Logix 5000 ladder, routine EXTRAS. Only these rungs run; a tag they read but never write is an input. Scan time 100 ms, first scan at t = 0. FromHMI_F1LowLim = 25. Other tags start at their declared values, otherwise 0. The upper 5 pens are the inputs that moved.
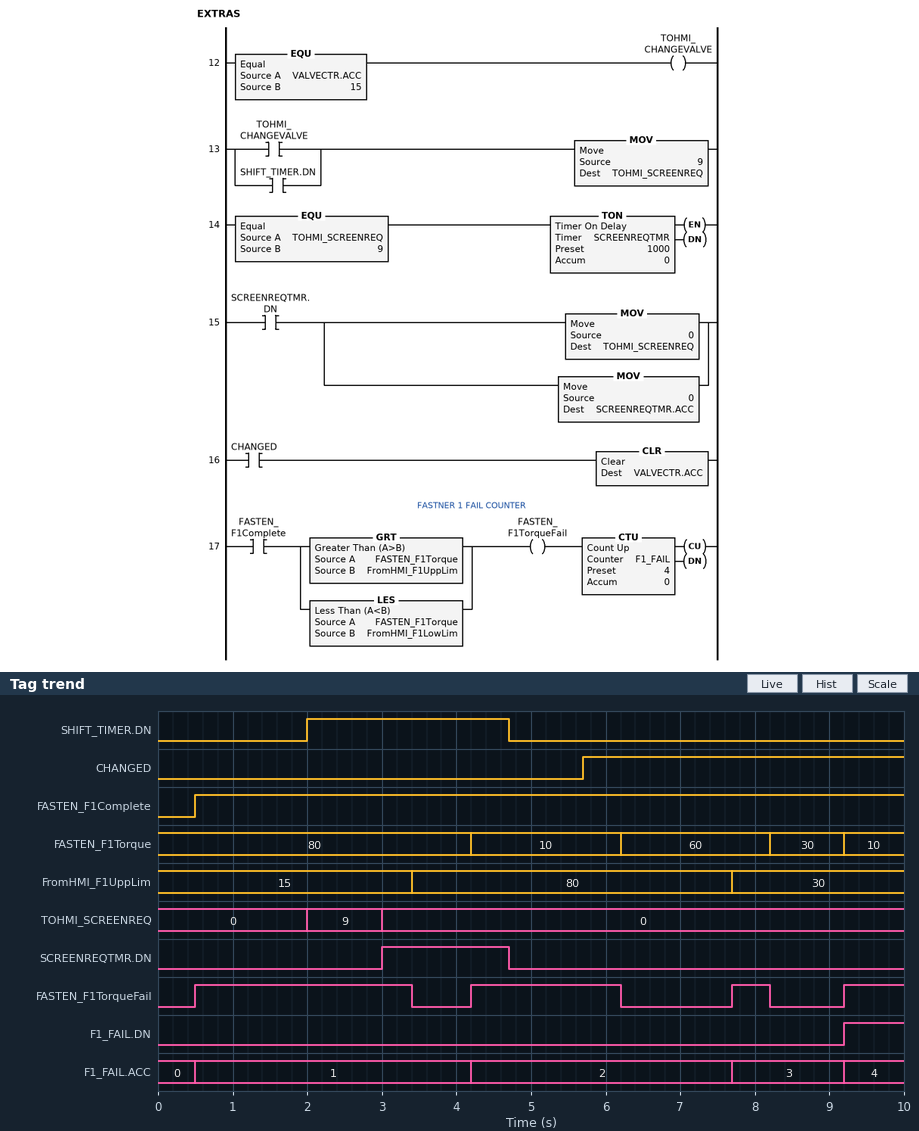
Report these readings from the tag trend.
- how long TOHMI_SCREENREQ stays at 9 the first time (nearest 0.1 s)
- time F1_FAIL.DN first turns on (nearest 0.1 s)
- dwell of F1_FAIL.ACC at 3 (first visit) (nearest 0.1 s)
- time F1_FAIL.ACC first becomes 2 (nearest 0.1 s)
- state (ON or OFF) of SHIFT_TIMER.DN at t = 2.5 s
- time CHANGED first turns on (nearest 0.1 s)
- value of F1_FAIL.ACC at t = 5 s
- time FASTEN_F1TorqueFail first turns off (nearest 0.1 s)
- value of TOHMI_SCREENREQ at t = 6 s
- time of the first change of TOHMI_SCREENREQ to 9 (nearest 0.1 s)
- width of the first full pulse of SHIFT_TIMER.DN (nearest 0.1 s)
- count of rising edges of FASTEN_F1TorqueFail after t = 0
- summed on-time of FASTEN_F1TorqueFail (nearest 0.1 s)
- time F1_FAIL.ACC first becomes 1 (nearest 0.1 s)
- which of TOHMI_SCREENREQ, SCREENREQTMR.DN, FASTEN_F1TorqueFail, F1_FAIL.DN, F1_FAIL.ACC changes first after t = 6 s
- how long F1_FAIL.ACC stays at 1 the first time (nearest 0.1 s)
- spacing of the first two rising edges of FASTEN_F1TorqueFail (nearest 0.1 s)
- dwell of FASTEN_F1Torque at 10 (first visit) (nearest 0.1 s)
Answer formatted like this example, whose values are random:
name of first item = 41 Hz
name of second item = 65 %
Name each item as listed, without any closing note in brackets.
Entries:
how long TOHMI_SCREENREQ stays at 9 the first time = 1.0 s
time F1_FAIL.DN first turns on = 9.2 s
dwell of F1_FAIL.ACC at 3 (first visit) = 1.5 s
time F1_FAIL.ACC first becomes 2 = 4.2 s
state (ON or OFF) of SHIFT_TIMER.DN at t = 2.5 s = ON
time CHANGED first turns on = 5.7 s
value of F1_FAIL.ACC at t = 5 s = 2
time FASTEN_F1TorqueFail first turns off = 3.4 s
value of TOHMI_SCREENREQ at t = 6 s = 0
time of the first change of TOHMI_SCREENREQ to 9 = 2.0 s
width of the first full pulse of SHIFT_TIMER.DN = 2.7 s
count of rising edges of FASTEN_F1TorqueFail after t = 0 = 4
summed on-time of FASTEN_F1TorqueFail = 6.2 s
time F1_FAIL.ACC first becomes 1 = 0.5 s
which of TOHMI_SCREENREQ, SCREENREQTMR.DN, FASTEN_F1TorqueFail, F1_FAIL.DN, F1_FAIL.ACC changes first after t = 6 s = FASTEN_F1TorqueFail
how long F1_FAIL.ACC stays at 1 the first time = 3.7 s
spacing of the first two rising edges of FASTEN_F1TorqueFail = 3.7 s
dwell of FASTEN_F1Torque at 10 (first visit) = 2.0 s
